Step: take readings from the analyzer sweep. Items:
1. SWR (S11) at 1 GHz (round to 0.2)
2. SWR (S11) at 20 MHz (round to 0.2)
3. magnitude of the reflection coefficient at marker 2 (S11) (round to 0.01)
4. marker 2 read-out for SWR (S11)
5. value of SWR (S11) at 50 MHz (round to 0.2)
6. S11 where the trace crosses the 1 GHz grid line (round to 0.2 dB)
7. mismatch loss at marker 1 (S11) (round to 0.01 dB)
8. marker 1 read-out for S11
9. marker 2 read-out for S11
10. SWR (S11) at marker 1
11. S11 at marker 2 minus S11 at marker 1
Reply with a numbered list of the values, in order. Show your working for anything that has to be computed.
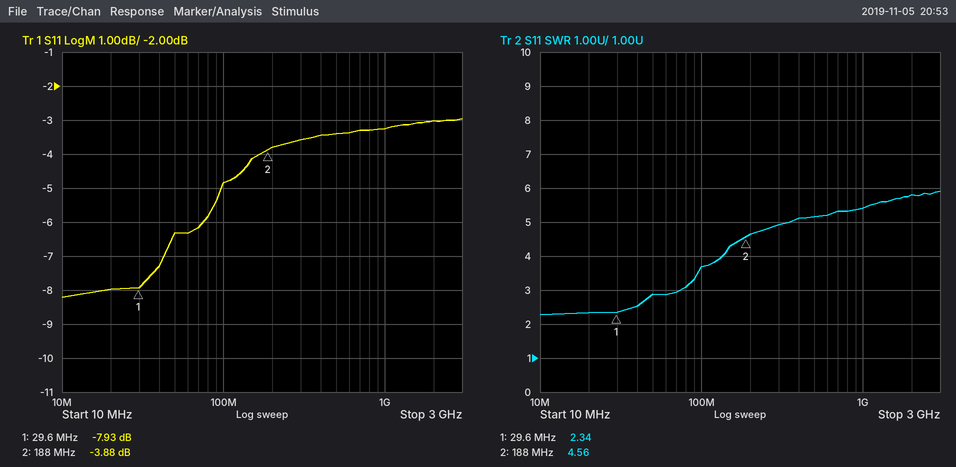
1. 5.4
2. 2.4
3. 10^(-3.88/20) ≈ 0.64
4. 4.56
5. 2.8
6. -3.2 dB
7. −10 log10(1 − 10^(-7.93/10)) ≈ 0.76 dB
8. -7.93 dB
9. -3.88 dB
10. 2.34
11. -3.88 − (-7.93) = 4.05 dB
